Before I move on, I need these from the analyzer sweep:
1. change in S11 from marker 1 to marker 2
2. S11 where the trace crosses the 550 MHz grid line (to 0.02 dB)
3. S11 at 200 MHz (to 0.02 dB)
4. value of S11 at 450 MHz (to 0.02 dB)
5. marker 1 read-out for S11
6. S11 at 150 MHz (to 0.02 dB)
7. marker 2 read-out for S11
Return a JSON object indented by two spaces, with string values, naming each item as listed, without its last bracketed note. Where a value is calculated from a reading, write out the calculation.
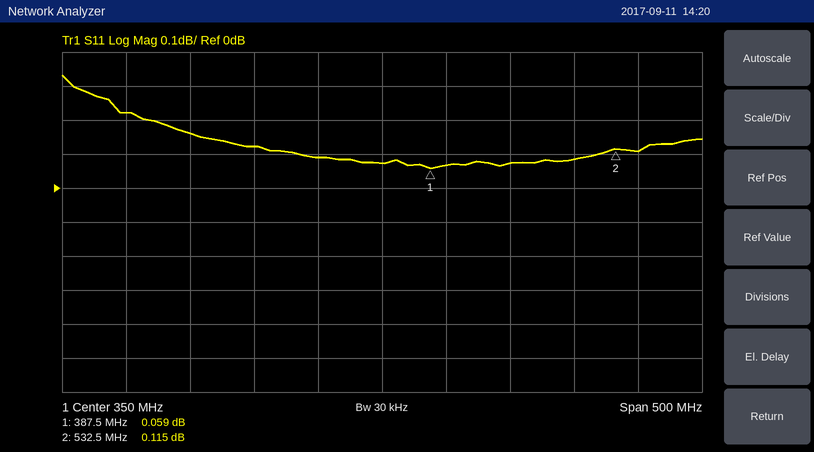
{
  "change in S11 from marker 1 to marker 2": "0.115 − (0.059) = 0.056 dB",
  "S11 where the trace crosses the 550 MHz grid line": "0.10 dB",
  "S11 at 200 MHz": "0.16 dB",
  "value of S11 at 450 MHz": "0.08 dB",
  "marker 1 read-out for S11": "0.059 dB",
  "S11 at 150 MHz": "0.22 dB",
  "marker 2 read-out for S11": "0.115 dB"
}
